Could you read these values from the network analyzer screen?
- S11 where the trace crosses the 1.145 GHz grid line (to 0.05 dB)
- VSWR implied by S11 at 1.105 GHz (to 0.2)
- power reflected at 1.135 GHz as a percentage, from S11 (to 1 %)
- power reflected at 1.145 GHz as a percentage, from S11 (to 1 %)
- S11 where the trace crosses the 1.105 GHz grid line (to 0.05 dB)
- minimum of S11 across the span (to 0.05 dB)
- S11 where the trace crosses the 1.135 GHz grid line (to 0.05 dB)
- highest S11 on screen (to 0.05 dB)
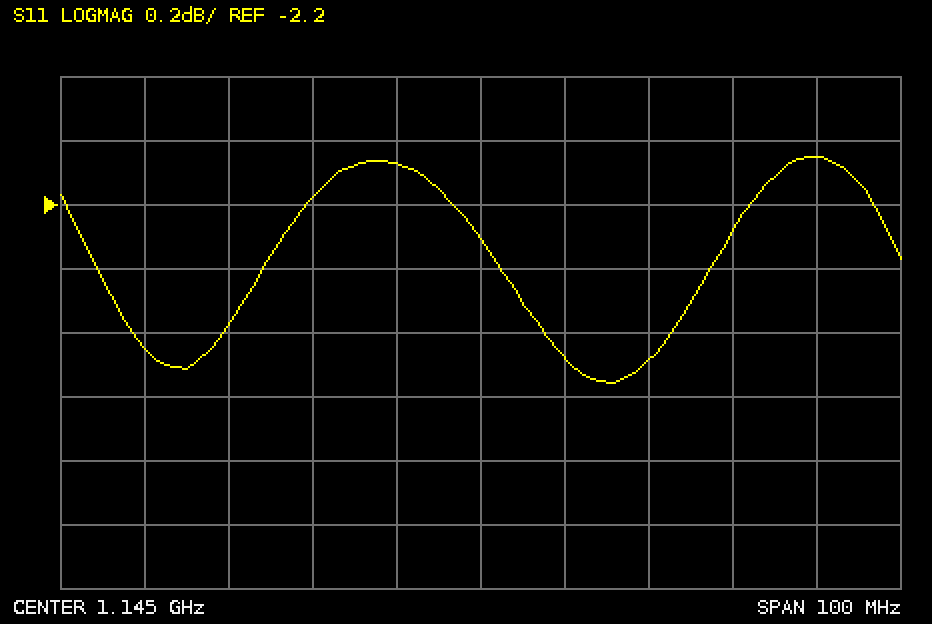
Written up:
-2.30 dB
6.6
62 %
59 %
-2.65 dB
-2.75 dB
-2.05 dB
-2.05 dB
